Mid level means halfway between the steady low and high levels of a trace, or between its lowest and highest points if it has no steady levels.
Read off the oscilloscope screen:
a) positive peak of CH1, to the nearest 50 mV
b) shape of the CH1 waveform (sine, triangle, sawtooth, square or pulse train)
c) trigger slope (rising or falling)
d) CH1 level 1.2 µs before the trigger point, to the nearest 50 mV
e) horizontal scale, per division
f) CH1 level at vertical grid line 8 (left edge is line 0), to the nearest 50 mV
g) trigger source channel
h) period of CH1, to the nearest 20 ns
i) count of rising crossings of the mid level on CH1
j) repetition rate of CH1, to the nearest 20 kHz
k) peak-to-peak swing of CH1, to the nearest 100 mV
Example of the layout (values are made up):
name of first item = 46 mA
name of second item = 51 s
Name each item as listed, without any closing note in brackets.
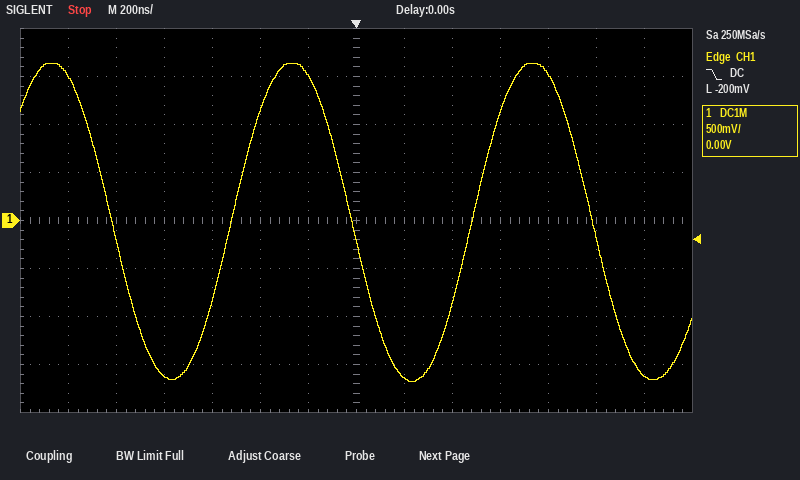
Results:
positive peak of CH1, to the nearest 50 mV = 1.65 V
shape of the CH1 waveform = sine
trigger slope = falling
CH1 level 1.2 µs before the trigger point, to the nearest 50 mV = 1.50 V
horizontal scale, per division = 200 ns
CH1 level at vertical grid line 8 (left edge is line 0), to the nearest 50 mV = -1.65 V
trigger source channel = CH1
period of CH1, to the nearest 20 ns = 1.00 µs
count of rising crossings of the mid level on CH1 = 2
repetition rate of CH1, to the nearest 20 kHz = 1.00 MHz
peak-to-peak swing of CH1, to the nearest 100 mV = 3.30 V
